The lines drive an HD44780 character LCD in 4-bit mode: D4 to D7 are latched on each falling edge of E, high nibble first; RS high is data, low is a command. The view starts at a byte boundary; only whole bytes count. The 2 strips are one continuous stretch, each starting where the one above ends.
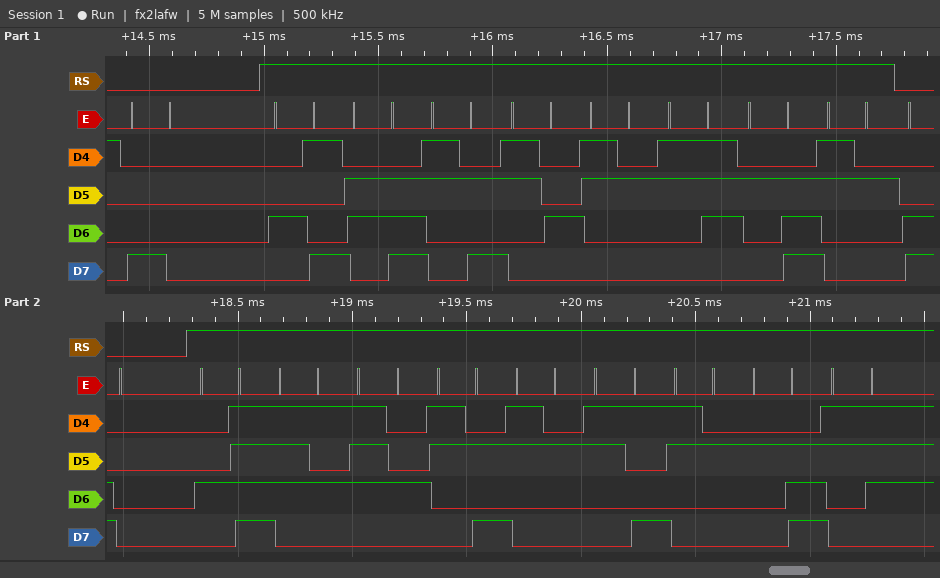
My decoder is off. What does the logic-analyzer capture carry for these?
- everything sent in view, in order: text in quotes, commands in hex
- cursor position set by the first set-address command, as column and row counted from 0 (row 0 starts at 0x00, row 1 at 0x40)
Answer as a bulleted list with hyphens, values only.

- 0x80 "In:427.2" 0xC0 "Out:292.7"
- column 0, row 0
